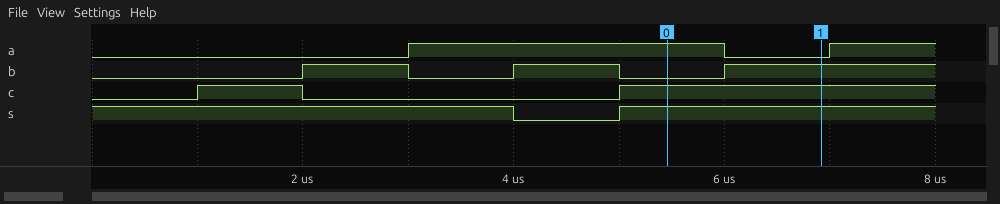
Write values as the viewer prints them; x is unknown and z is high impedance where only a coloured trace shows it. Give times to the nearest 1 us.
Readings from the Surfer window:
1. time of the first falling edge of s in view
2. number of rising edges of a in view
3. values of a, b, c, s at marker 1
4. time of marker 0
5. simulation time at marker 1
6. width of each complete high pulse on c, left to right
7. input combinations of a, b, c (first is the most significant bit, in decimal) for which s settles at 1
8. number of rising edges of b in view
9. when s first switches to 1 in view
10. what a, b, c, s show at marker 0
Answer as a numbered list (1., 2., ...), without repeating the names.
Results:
1. 4 us
2. 2
3. a=0, b=1, c=1, s=1
4. 5 us
5. 7 us
6. 1 us
7. 0, 1, 2, 3, 4, 5, 7
8. 3
9. 5 us
10. a=1, b=0, c=1, s=1
